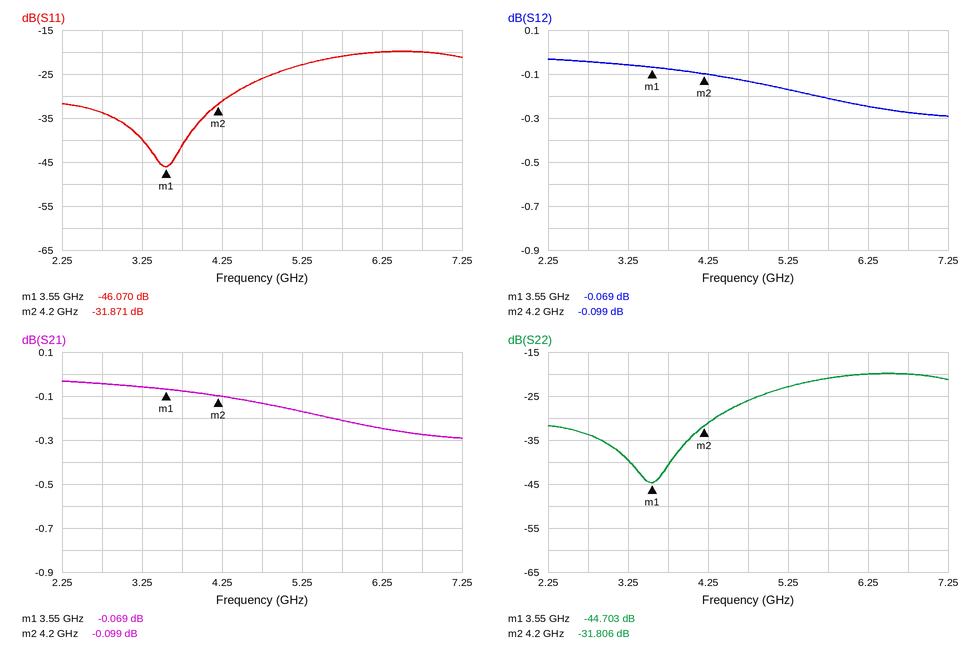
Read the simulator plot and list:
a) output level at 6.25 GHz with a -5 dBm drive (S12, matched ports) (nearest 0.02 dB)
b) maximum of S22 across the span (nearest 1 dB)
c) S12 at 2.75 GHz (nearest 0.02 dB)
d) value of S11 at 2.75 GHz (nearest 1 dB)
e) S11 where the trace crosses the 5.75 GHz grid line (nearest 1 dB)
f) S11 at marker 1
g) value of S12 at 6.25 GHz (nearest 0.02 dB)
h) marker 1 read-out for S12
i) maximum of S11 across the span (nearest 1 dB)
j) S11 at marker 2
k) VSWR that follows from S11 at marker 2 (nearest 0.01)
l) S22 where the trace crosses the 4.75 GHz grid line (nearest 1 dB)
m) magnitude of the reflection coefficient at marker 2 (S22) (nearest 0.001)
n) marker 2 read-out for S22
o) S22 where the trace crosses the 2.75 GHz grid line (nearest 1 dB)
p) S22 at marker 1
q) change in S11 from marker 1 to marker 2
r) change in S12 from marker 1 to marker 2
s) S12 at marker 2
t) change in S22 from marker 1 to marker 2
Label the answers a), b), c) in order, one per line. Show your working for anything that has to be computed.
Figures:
a) -5 dBm + (-0.24 dB) = -5.24 dBm
b) -20 dB
c) -0.04 dB
d) -34 dB
e) -21 dB
f) -46.070 dB
g) -0.24 dB
h) -0.069 dB
i) -20 dB
j) -31.871 dB
k) (1 + 0.0255)/(1 − 0.0255) ≈ 1.05
l) -26 dB
m) 10^(-31.806/20) ≈ 0.026
n) -31.806 dB
o) -34 dB
p) -44.703 dB
q) -31.871 − (-46.07) = 14.199 dB
r) -0.099 − (-0.069) = -0.030 dB
s) -0.099 dB
t) -31.806 − (-44.703) = 12.897 dB
